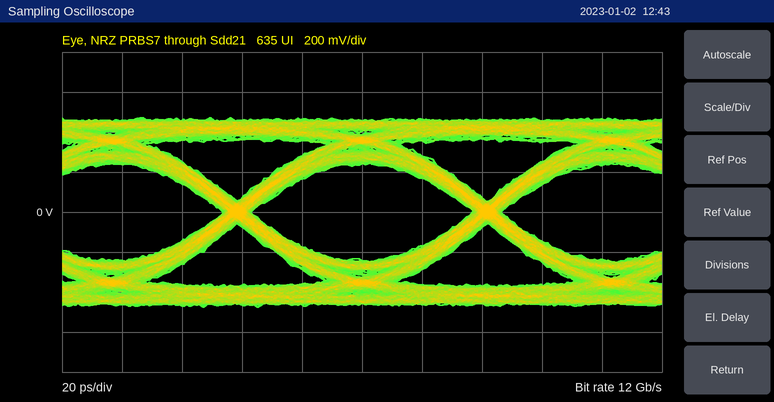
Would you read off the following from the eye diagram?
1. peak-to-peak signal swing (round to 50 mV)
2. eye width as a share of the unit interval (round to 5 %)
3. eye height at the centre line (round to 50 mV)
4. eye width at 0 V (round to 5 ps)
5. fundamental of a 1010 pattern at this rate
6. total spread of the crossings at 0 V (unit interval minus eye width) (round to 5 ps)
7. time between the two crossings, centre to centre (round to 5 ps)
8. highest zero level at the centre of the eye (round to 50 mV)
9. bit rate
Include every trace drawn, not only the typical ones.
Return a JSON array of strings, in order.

["950 mV", "90 %", "500 mV", "75 ps", "6 GHz", "10 ps", "85 ps", "-250 mV", "12 Gb/s"]
